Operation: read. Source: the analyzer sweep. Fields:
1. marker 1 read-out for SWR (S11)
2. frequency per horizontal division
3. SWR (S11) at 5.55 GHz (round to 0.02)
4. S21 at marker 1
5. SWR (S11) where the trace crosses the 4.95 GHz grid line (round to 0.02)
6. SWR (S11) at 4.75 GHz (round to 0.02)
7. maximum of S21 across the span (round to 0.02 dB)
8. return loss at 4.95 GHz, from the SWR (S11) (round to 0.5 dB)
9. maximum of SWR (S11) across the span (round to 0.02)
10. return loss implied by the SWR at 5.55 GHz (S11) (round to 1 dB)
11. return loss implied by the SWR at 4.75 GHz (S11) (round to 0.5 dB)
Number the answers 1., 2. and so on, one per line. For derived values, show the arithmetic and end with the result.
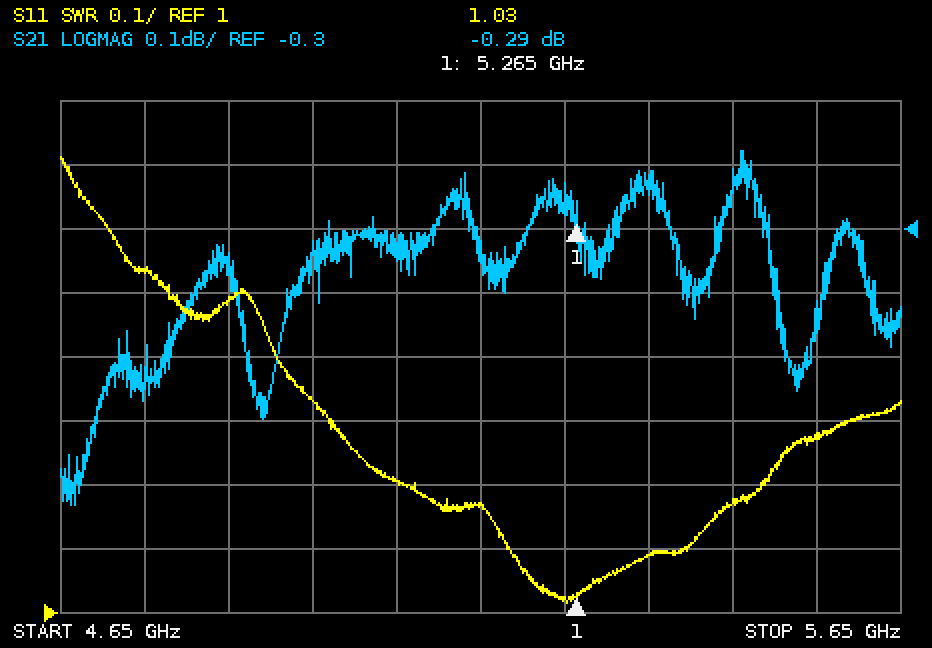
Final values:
1. 1.03
2. 100 MHz
3. 1.28
4. -0.29 dB
5. 1.34
6. 1.54
7. -0.18 dB
8. −20 log10((1.34 − 1)/(1.34 + 1)) ≈ 16.8 dB, so 17.0 dB to the nearest 0.5 dB
9. 1.72
10. −20 log10((1.28 − 1)/(1.28 + 1)) ≈ 18 dB
11. −20 log10((1.54 − 1)/(1.54 + 1)) ≈ 13.4 dB, so 13.5 dB to the nearest 0.5 dB
